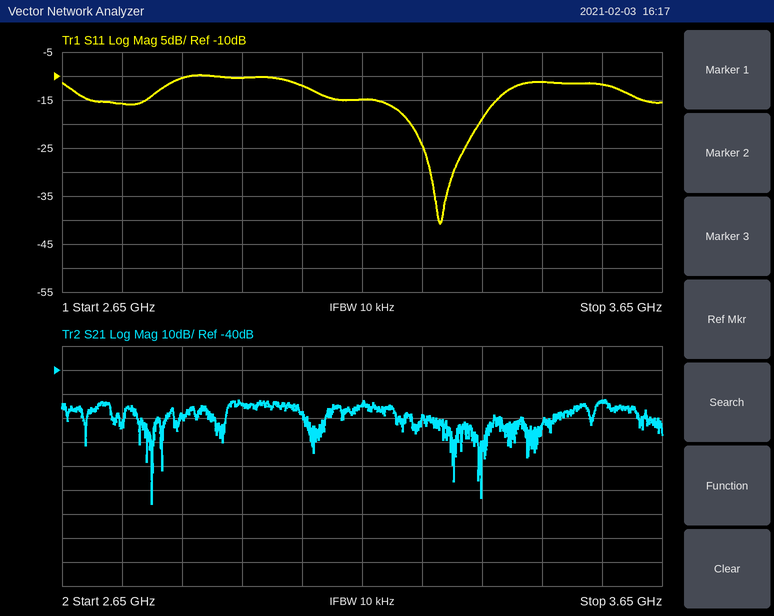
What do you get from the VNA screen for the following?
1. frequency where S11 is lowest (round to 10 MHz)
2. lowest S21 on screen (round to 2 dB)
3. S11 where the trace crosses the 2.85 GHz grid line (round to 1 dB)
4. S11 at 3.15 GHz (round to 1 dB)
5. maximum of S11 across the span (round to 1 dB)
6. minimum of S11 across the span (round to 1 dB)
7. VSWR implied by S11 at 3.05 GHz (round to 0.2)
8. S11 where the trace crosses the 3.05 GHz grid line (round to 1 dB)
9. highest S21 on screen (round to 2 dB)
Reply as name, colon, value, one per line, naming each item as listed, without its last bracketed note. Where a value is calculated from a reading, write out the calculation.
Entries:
frequency where S11 is lowest: 3.28 GHz
lowest S21 on screen: -96 dB
S11 where the trace crosses the 2.85 GHz grid line: -10 dB
S11 at 3.15 GHz: -15 dB
maximum of S11 across the span: -10 dB
minimum of S11 across the span: -41 dB
VSWR implied by S11 at 3.05 GHz: |Γ| = 10^(-12/20) = 0.2512; VSWR = (1 + 0.2512)/(1 − 0.2512) ≈ 1.67, so 1.6 to the nearest 0.2
S11 where the trace crosses the 3.05 GHz grid line: -12 dB
highest S21 on screen: -52 dB
